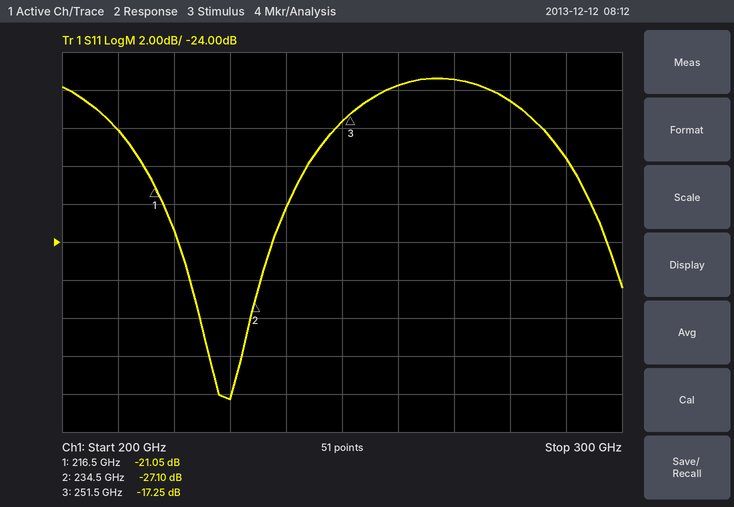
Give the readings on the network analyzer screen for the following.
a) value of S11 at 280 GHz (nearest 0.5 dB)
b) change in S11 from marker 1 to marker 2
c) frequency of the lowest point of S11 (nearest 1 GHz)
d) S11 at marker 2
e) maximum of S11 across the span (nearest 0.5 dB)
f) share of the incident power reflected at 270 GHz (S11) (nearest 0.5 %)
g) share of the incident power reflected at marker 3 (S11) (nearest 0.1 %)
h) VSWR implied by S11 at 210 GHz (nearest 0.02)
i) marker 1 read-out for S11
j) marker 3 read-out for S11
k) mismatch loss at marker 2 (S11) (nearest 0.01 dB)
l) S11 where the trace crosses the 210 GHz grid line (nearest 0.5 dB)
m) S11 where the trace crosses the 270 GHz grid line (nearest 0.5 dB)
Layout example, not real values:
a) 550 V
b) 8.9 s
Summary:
a) -16.5 dB
b) -6.05 dB
c) 230 GHz
d) -27.10 dB
e) -15.5 dB
f) 3.0 %
g) 1.9 %
h) 1.28
i) -21.05 dB
j) -17.25 dB
k) 0.01 dB
l) -18.0 dB
m) -15.5 dB
